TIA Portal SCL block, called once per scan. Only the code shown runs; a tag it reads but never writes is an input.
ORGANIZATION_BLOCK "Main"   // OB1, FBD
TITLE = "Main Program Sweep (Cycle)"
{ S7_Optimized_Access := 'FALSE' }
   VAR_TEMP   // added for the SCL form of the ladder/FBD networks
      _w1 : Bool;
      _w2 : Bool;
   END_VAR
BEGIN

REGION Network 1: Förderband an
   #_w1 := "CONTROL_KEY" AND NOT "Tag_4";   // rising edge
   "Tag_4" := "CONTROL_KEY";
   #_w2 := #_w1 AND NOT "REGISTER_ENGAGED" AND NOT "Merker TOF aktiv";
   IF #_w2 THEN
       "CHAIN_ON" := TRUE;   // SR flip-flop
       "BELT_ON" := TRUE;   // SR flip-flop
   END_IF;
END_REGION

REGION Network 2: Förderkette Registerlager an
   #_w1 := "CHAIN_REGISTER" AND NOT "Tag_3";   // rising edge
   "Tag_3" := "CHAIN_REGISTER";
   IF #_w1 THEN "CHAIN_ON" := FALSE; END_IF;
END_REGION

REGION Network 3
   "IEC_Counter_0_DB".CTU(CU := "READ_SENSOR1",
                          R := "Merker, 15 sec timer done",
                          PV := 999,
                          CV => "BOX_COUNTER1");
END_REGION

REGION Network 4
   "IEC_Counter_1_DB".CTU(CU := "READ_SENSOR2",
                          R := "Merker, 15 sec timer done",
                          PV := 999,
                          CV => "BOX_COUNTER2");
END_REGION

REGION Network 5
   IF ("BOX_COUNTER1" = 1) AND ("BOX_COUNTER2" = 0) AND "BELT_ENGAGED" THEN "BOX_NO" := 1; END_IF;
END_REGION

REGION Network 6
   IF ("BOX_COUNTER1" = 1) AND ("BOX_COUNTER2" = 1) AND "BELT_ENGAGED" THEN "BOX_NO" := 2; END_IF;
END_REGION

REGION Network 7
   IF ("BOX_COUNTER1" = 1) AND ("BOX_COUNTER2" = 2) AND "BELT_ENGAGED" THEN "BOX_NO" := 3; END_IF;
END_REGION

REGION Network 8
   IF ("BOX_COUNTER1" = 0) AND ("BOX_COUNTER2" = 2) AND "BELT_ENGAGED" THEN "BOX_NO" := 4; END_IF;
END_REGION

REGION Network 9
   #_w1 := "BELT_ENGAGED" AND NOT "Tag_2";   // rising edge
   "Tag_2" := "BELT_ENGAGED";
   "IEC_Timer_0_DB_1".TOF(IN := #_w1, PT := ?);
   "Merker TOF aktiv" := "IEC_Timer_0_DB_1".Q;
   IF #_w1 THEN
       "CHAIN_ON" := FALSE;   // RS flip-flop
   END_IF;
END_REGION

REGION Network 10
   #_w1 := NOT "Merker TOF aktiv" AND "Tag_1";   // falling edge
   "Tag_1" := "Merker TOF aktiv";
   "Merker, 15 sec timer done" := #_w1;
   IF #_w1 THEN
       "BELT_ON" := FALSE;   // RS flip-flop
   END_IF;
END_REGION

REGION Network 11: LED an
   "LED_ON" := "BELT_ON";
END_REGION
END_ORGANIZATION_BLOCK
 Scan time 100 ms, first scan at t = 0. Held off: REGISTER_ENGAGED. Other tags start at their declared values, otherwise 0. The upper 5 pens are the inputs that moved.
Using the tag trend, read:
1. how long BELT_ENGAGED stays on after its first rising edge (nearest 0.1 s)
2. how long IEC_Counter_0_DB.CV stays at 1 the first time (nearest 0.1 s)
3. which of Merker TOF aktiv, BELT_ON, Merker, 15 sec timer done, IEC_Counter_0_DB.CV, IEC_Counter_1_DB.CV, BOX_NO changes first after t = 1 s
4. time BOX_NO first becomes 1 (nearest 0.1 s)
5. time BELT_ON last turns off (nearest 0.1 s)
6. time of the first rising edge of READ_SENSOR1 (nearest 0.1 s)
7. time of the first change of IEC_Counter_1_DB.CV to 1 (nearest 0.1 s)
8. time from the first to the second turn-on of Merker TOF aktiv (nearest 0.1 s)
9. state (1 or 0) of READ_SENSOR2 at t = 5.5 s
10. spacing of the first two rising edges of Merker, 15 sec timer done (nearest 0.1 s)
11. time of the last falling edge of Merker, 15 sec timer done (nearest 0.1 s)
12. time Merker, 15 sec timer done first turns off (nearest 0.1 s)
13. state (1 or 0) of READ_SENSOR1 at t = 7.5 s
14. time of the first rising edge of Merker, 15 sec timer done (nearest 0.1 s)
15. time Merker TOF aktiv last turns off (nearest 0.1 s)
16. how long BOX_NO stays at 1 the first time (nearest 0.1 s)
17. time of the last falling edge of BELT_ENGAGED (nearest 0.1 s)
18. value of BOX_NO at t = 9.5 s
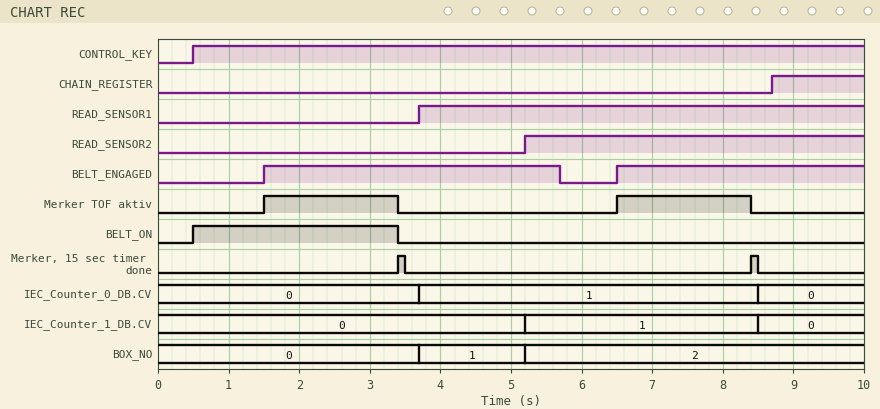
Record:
4.2 s
4.8 s
Merker TOF aktiv
3.7 s
3.4 s
3.7 s
5.2 s
5.0 s
1
5.0 s
8.5 s
3.5 s
1
3.4 s
8.4 s
1.5 s
5.7 s
2
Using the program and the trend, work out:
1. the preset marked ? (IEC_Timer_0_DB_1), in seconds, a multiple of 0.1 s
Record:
1.8 s
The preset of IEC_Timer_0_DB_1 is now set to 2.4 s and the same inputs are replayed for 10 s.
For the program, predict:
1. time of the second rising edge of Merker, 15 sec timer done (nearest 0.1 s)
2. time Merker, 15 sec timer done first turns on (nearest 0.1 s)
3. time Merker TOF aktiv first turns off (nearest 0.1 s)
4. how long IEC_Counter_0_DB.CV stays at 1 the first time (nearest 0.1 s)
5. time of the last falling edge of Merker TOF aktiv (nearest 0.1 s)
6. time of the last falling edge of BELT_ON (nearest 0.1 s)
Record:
9.0 s
4.0 s
4.0 s
0.4 s
9.0 s
4.0 s
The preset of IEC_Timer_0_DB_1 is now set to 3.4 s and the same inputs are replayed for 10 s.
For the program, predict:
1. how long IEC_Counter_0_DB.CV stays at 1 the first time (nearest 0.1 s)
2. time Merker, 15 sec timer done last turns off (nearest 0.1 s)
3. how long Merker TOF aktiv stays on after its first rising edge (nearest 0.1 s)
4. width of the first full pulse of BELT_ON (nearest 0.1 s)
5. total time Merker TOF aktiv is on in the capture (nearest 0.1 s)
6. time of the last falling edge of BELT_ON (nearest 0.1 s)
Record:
1.4 s
5.1 s
3.5 s
4.5 s
7.0 s
5.0 s
